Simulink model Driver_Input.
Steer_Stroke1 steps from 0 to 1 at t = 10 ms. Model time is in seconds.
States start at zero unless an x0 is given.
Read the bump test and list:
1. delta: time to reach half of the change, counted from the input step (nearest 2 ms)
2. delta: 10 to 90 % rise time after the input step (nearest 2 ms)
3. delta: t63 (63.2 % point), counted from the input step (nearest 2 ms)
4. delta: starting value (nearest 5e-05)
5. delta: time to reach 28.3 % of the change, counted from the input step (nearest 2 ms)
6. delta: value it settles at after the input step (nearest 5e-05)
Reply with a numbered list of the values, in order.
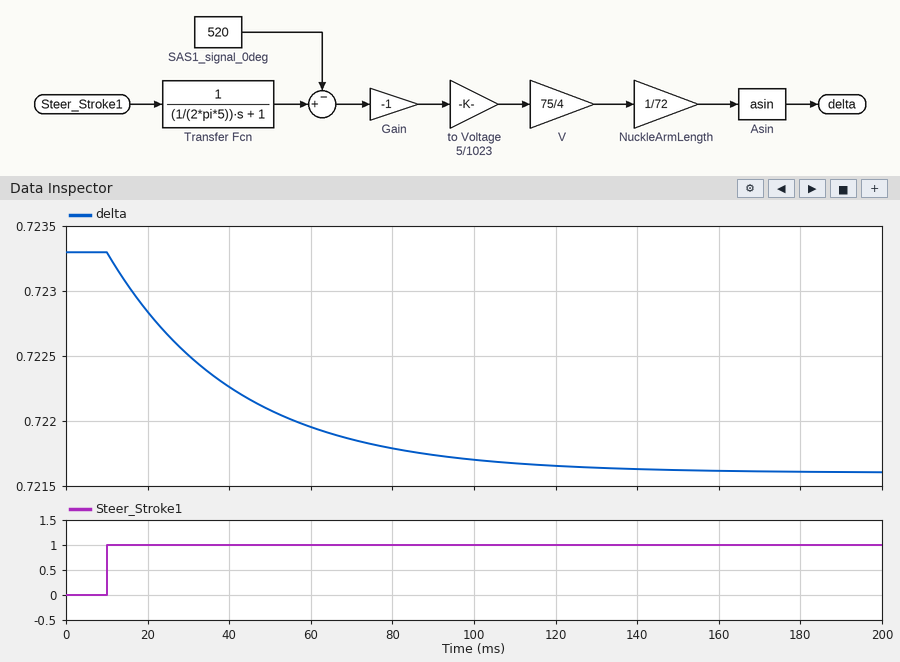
1. 22 ms
2. 70 ms
3. 32 ms
4. 0.72330
5. 10 ms
6. 0.72160
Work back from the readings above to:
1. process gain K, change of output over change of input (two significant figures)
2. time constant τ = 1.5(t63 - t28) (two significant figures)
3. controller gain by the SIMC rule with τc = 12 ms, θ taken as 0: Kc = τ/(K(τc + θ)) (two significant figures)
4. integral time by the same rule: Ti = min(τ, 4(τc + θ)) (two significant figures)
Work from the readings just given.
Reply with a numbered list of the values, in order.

1. -0.0017
2. 33 ms
3. -1600
4. 33 ms
